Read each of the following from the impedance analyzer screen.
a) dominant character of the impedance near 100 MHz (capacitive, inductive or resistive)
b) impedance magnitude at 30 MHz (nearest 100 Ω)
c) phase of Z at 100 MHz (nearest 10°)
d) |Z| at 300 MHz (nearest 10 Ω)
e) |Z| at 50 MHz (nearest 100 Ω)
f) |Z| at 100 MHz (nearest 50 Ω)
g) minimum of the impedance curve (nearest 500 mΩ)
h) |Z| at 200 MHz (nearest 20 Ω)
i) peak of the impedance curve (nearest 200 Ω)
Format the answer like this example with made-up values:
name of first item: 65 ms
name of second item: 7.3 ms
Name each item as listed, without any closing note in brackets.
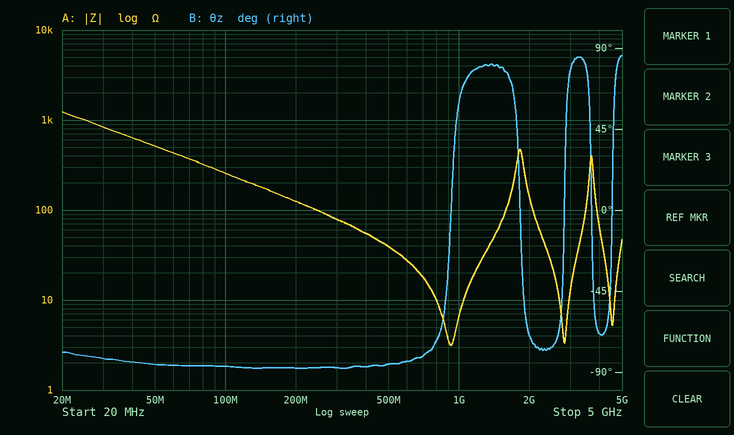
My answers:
dominant character of the impedance near 100 MHz: capacitive
impedance magnitude at 30 MHz: 800 Ω
phase of Z at 100 MHz: -90°
|Z| at 300 MHz: 80 Ω
|Z| at 50 MHz: 500 Ω
|Z| at 100 MHz: 250 Ω
minimum of the impedance curve: 3.0 Ω
|Z| at 200 MHz: 120 Ω
peak of the impedance curve: 1.2 kΩ
